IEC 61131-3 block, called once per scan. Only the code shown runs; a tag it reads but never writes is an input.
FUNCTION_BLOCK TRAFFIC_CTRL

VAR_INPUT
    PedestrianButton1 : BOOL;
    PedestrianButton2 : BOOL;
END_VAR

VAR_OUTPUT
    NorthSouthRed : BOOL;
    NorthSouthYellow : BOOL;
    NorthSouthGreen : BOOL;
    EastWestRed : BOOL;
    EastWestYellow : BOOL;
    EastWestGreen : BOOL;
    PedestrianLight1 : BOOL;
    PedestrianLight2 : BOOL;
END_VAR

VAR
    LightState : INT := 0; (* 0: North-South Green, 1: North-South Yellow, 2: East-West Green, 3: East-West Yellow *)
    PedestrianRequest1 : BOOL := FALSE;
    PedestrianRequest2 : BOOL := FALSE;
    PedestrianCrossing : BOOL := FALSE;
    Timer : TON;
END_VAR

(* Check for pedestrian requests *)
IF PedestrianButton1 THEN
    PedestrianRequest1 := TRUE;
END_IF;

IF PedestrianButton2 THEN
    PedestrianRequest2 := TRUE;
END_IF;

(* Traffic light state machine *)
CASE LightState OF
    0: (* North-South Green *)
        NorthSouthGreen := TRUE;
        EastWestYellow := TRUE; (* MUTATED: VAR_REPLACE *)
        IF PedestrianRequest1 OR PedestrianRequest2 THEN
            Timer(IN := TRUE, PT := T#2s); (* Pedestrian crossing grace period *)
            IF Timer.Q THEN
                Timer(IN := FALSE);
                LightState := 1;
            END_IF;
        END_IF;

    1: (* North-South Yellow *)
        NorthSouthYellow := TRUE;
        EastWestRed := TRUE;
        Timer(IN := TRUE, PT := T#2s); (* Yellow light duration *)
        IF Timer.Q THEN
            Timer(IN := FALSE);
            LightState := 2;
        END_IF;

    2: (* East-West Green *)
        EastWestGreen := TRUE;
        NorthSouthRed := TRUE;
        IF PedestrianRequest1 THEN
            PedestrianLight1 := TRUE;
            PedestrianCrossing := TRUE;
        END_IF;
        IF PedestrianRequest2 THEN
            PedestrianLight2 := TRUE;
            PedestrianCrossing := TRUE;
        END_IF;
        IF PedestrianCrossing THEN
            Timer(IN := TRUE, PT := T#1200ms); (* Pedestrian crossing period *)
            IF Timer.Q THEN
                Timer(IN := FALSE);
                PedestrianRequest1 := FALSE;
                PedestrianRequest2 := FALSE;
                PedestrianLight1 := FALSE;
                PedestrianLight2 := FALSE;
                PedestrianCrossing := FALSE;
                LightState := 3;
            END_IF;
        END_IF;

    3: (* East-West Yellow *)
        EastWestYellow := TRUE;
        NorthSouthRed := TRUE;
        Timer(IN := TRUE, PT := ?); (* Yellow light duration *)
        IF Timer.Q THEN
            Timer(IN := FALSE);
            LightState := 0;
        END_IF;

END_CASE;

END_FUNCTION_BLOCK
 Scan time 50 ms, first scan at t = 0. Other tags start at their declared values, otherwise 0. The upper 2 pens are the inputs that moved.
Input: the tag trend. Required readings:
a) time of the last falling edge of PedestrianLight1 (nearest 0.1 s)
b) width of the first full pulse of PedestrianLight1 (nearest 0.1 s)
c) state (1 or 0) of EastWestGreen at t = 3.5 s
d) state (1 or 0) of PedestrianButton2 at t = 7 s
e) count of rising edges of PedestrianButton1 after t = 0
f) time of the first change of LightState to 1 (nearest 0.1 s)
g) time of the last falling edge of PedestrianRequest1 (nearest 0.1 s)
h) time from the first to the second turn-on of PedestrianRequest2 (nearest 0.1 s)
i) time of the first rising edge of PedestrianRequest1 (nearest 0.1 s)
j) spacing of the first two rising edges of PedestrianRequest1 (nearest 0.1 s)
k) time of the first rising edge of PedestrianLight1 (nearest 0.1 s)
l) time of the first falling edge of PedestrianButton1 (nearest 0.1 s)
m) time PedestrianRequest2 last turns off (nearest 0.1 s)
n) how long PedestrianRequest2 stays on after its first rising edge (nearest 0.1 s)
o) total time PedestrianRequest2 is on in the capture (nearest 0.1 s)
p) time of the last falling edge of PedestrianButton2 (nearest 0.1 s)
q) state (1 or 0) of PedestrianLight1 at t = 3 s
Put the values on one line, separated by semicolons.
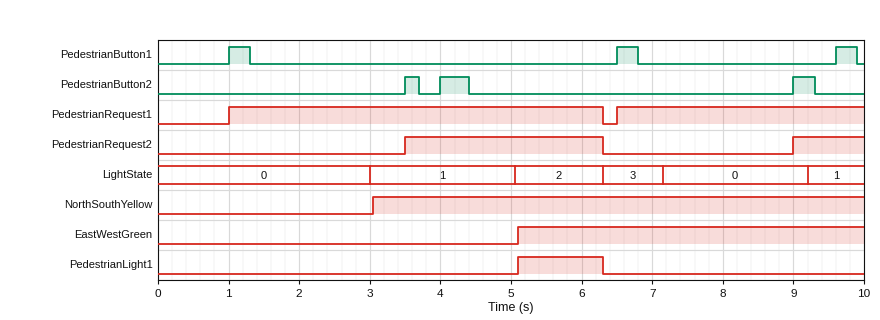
6.3 s; 1.2 s; 0; 0; 3; 3.0 s; 6.3 s; 5.5 s; 1.0 s; 5.5 s; 5.1 s; 1.3 s; 6.3 s; 2.8 s; 3.8 s; 9.3 s; 0
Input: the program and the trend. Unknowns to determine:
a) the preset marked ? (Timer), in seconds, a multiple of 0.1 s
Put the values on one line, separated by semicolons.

0.8 s
